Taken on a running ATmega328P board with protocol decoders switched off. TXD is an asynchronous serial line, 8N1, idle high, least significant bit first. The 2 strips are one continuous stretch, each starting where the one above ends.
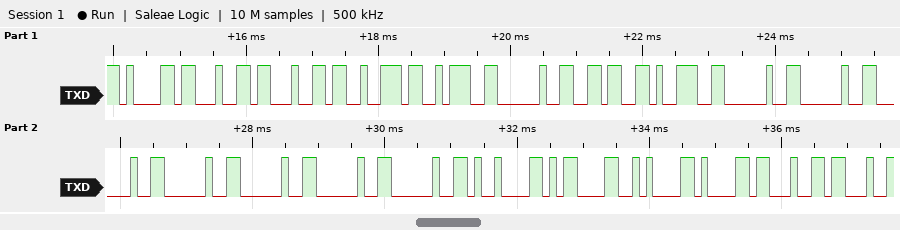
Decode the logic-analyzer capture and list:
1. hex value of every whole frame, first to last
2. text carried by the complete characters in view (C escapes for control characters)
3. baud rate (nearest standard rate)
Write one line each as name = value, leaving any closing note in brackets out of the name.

hex value of every whole frame, first to last = 61 64 64 72 3A 20 36 39 20 20 20 20 20 20 20 09 0D 0A 61 64
text carried by the complete characters in view = "addr: 69       \t\r\nad"
baud rate = 9600 baud
